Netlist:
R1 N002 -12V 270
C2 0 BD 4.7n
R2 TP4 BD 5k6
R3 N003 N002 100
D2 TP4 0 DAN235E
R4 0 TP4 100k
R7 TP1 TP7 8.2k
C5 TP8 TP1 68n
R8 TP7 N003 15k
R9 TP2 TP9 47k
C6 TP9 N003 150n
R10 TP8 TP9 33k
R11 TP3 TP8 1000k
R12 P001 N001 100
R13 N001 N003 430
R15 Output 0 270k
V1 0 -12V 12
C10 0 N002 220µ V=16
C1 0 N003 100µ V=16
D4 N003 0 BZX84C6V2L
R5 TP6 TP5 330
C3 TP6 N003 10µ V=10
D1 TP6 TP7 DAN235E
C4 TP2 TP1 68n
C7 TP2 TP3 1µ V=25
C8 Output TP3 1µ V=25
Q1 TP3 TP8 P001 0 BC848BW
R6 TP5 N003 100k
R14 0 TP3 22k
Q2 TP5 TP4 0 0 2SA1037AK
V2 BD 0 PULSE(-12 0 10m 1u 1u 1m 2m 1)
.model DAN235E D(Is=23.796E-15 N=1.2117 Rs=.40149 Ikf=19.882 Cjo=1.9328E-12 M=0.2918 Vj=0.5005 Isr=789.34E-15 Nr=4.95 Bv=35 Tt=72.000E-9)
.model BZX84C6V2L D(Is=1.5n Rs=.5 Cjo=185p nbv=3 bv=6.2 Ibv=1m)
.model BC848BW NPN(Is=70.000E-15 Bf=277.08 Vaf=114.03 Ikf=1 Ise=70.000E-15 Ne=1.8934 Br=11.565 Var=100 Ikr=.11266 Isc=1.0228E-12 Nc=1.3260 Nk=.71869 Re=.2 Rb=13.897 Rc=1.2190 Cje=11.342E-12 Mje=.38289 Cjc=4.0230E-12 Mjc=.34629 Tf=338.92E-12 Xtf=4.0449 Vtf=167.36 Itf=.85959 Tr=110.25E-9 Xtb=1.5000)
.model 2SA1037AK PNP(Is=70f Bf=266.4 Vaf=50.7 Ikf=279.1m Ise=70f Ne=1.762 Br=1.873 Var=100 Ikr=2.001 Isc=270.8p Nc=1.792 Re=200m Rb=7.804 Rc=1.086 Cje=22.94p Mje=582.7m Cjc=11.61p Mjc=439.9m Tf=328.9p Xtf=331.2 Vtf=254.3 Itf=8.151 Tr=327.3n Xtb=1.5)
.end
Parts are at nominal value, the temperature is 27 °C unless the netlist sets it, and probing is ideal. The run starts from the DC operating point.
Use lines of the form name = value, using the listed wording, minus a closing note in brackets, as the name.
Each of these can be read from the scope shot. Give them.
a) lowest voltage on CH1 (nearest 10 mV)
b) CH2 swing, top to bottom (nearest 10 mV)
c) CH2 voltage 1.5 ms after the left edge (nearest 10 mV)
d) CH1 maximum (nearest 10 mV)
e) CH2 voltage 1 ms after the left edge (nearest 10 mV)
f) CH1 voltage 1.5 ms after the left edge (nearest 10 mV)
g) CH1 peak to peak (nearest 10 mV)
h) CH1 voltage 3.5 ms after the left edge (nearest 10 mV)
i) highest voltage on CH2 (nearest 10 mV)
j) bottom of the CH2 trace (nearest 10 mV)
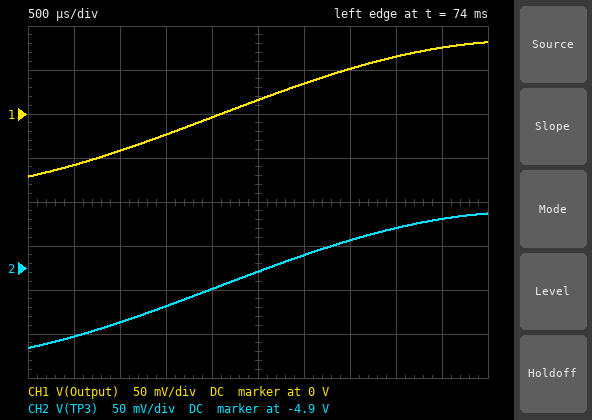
lowest voltage on CH1 = -70 mV
CH2 swing, top to bottom = 150 mV
CH2 voltage 1.5 ms after the left edge = -4.94 V
CH1 maximum = 80 mV
CH2 voltage 1 ms after the left edge = -4.96 V
CH1 voltage 1.5 ms after the left edge = -20 mV
CH1 peak to peak = 150 mV
CH1 voltage 3.5 ms after the left edge = 50 mV
highest voltage on CH2 = -4.84 V
bottom of the CH2 trace = -4.99 V
